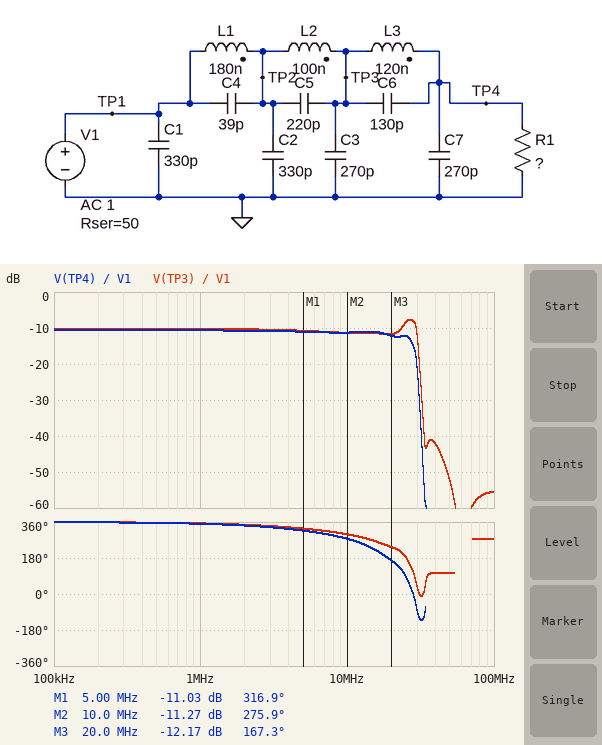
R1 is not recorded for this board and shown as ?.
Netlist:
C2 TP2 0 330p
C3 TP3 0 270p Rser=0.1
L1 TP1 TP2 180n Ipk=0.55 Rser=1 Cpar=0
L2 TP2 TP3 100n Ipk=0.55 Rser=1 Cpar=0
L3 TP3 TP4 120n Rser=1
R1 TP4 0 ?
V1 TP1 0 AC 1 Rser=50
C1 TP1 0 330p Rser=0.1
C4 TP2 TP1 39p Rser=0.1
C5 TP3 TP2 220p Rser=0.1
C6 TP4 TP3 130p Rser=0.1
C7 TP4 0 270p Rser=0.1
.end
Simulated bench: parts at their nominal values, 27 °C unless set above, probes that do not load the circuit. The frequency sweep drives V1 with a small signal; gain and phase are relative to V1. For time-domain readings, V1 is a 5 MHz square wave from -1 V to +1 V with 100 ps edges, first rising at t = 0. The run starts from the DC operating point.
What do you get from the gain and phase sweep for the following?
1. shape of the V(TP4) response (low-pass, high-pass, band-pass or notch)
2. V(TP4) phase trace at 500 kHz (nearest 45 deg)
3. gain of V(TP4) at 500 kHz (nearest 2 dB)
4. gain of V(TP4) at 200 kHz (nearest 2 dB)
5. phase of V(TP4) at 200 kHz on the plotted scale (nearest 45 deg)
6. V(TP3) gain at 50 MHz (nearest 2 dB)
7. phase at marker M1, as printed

low-pass
360 deg
-10 dB
-10 dB
360 deg
-52 dB
316.9 deg
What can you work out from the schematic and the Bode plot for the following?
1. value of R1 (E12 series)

22 Ω
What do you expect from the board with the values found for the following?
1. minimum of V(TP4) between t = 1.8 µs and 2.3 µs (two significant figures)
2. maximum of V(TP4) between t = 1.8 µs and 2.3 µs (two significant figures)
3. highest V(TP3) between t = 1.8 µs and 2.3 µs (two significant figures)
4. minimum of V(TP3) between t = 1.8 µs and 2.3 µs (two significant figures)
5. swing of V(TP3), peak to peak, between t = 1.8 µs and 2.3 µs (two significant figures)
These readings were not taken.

-380 mV
380 mV
360 mV
-360 mV
720 mV
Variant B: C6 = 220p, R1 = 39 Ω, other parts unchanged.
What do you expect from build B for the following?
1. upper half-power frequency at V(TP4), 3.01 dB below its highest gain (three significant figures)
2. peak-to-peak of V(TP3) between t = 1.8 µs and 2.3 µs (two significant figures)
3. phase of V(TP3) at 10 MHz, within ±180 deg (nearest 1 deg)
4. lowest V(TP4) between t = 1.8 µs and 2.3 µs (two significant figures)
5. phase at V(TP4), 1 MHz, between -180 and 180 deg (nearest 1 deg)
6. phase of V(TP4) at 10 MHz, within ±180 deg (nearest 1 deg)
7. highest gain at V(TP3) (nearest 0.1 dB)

23.9 MHz
940 mV
-72 deg
-450 mV
-11 deg
-87 deg
-6.0 dB
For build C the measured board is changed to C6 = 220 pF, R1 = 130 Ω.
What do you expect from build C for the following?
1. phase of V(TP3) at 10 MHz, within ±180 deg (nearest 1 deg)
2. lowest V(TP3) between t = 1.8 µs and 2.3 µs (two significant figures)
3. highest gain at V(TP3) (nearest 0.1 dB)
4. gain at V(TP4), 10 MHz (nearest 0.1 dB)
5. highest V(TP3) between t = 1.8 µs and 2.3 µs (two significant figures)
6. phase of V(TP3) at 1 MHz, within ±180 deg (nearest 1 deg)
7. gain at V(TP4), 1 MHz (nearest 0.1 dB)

-84 deg
-670 mV
-2.9 dB
-8.5 dB
670 mV
-16 deg
-3.2 dB
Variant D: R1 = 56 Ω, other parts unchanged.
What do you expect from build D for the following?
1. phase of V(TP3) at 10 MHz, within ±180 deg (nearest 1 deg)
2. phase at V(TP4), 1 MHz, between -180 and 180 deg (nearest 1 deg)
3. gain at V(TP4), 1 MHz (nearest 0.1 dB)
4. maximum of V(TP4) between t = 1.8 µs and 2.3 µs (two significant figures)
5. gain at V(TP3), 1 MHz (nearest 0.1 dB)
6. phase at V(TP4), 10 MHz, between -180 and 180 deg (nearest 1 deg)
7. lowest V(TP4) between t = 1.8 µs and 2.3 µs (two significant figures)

-77 deg
-13 deg
-5.9 dB
480 mV
-5.8 dB
-88 deg
-480 mV
